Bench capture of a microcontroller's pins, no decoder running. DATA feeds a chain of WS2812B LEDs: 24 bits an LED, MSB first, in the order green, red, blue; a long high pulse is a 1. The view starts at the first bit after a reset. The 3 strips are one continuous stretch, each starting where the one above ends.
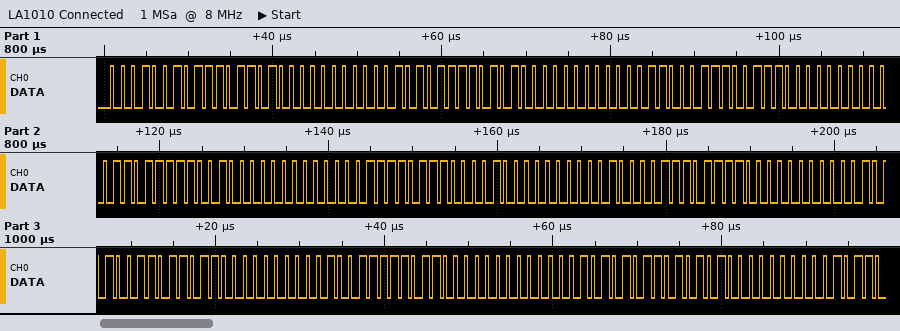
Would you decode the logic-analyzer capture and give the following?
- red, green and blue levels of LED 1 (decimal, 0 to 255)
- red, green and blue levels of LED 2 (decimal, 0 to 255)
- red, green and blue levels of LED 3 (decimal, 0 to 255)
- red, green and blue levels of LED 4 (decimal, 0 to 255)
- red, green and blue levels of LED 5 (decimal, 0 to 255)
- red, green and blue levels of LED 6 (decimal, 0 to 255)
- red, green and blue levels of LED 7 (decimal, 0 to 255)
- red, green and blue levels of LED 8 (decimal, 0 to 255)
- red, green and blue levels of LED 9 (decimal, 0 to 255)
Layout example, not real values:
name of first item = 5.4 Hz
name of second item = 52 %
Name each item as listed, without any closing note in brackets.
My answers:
red, green and blue levels of LED 1 = 237, 18, 0
red, green and blue levels of LED 2 = 234, 21, 0
red, green and blue levels of LED 3 = 231, 24, 0
red, green and blue levels of LED 4 = 228, 27, 0
red, green and blue levels of LED 5 = 225, 30, 0
red, green and blue levels of LED 6 = 222, 33, 0
red, green and blue levels of LED 7 = 219, 36, 0
red, green and blue levels of LED 8 = 216, 39, 0
red, green and blue levels of LED 9 = 213, 42, 0
